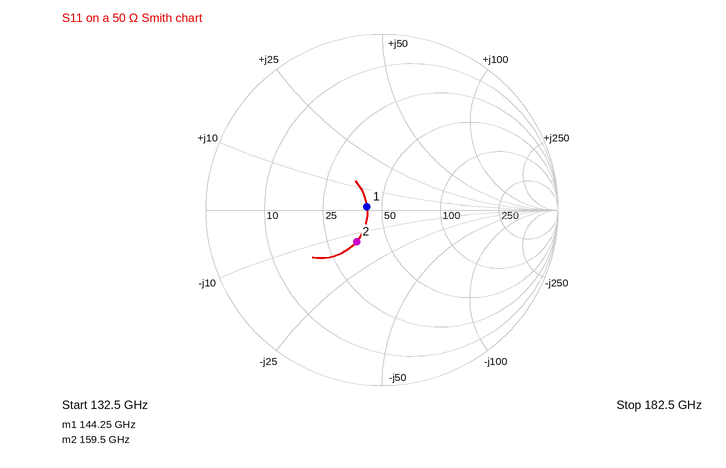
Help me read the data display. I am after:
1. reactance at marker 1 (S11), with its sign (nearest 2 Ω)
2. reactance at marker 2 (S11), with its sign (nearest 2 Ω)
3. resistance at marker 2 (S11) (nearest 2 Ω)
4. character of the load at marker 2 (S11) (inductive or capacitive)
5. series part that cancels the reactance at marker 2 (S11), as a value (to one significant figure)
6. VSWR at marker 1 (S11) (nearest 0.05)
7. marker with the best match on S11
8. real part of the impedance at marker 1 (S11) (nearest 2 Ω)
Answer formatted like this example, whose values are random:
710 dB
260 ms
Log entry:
+2 Ω
-14 Ω
36 Ω
capacitive
10 pH
1.20
marker 1
42 Ω
